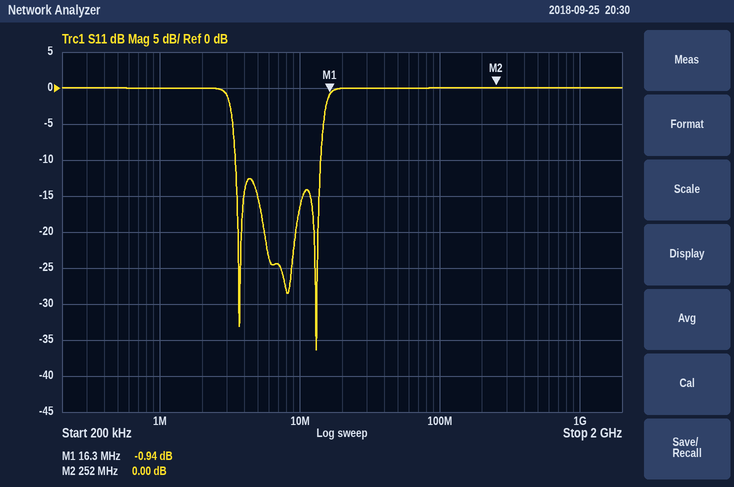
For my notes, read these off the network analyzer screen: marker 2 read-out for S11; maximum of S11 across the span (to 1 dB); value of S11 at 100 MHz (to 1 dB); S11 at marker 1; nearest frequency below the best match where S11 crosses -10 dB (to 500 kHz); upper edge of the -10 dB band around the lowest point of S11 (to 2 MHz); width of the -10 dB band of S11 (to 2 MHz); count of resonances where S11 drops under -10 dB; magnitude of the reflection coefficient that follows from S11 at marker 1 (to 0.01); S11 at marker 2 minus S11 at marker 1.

0.00 dB
0 dB
0 dB
-0.94 dB
3.5 MHz
14 MHz
10 MHz
3
0.90
0.94 dB
